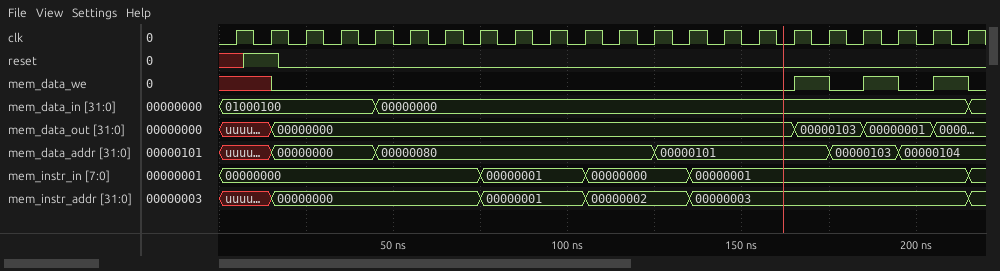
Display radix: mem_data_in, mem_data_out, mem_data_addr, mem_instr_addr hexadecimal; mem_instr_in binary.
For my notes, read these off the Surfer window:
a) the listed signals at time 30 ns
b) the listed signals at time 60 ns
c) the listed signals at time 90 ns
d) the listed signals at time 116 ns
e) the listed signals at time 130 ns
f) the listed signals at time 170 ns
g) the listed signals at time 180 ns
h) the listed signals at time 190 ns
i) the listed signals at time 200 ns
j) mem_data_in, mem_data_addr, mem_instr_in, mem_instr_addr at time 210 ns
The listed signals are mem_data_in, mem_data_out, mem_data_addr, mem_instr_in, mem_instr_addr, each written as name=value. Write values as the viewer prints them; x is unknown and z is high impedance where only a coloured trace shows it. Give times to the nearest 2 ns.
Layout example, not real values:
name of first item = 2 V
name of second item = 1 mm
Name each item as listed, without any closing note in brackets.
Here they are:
the listed signals at time 30 ns = mem_data_in=01000100, mem_data_out=00000000, mem_data_addr=00000000, mem_instr_in=00000000, mem_instr_addr=00000000
the listed signals at time 60 ns = mem_data_in=00000000, mem_data_out=00000000, mem_data_addr=00000080, mem_instr_in=00000000, mem_instr_addr=00000000
the listed signals at time 90 ns = mem_data_in=00000000, mem_data_out=00000000, mem_data_addr=00000080, mem_instr_in=00000001, mem_instr_addr=00000001
the listed signals at time 116 ns = mem_data_in=00000000, mem_data_out=00000000, mem_data_addr=00000080, mem_instr_in=00000000, mem_instr_addr=00000002
the listed signals at time 130 ns = mem_data_in=00000000, mem_data_out=00000000, mem_data_addr=00000101, mem_instr_in=00000000, mem_instr_addr=00000002
the listed signals at time 170 ns = mem_data_in=00000000, mem_data_out=00000103, mem_data_addr=00000101, mem_instr_in=00000001, mem_instr_addr=00000003
the listed signals at time 180 ns = mem_data_in=00000000, mem_data_out=00000103, mem_data_addr=00000103, mem_instr_in=00000001, mem_instr_addr=00000003
the listed signals at time 190 ns = mem_data_in=00000000, mem_data_out=00000001, mem_data_addr=00000103, mem_instr_in=00000001, mem_instr_addr=00000003
the listed signals at time 200 ns = mem_data_in=00000000, mem_data_out=00000001, mem_data_addr=00000104, mem_instr_in=00000001, mem_instr_addr=00000003
mem_data_in, mem_data_addr, mem_instr_in, mem_instr_addr at time 210 ns = mem_data_in=00000000, mem_data_addr=00000104, mem_instr_in=00000001, mem_instr_addr=00000003
